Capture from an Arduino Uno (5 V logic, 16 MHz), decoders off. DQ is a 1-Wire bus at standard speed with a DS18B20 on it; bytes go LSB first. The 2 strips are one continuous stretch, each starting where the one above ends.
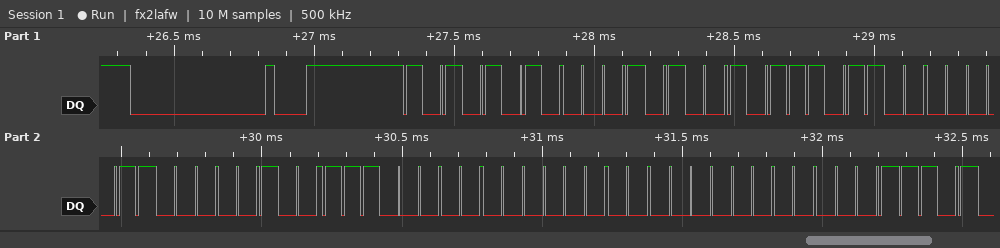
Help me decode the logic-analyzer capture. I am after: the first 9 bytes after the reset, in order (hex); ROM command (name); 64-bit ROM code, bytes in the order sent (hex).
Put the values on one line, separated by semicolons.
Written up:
55 28 DD C0 20 07 00 00 B8; Match ROM; 28 DD C0 20 07 00 00 B8
